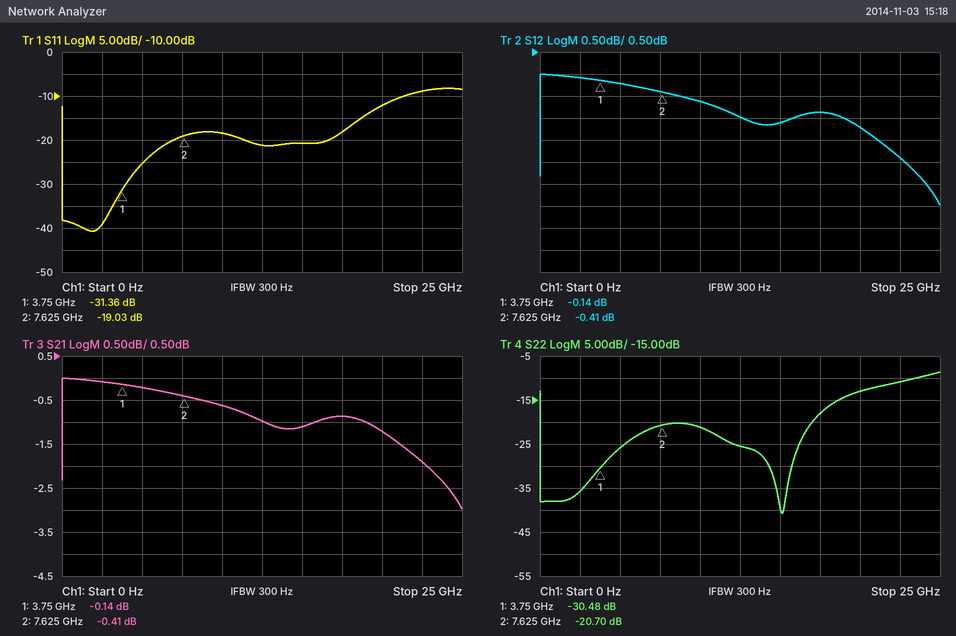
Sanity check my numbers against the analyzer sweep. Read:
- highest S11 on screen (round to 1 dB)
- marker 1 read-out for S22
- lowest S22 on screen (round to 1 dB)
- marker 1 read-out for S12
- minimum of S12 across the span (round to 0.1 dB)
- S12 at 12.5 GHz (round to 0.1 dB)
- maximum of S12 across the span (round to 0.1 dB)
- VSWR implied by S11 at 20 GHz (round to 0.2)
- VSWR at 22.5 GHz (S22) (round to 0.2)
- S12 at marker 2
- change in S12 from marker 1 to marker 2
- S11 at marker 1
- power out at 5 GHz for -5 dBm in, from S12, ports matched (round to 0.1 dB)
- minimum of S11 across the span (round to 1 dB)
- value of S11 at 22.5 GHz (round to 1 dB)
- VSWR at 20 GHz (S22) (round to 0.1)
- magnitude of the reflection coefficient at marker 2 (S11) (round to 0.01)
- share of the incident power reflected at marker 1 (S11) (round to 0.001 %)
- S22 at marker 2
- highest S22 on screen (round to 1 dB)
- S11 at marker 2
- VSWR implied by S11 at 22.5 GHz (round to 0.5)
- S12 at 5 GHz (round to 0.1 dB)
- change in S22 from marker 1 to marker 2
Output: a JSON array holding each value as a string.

["-8 dB", "-30.48 dB", "-41 dB", "-0.14 dB", "-3.0 dB", "-1.0 dB", "0.0 dB", "1.6", "1.8", "-0.41 dB", "-0.27 dB", "-31.36 dB", "-5.2 dBm", "-41 dB", "-9 dB", "1.6", "0.11", "0.073 %", "-20.70 dB", "-9 dB", "-19.03 dB", "2.0", "-0.2 dB", "9.78 dB"]
